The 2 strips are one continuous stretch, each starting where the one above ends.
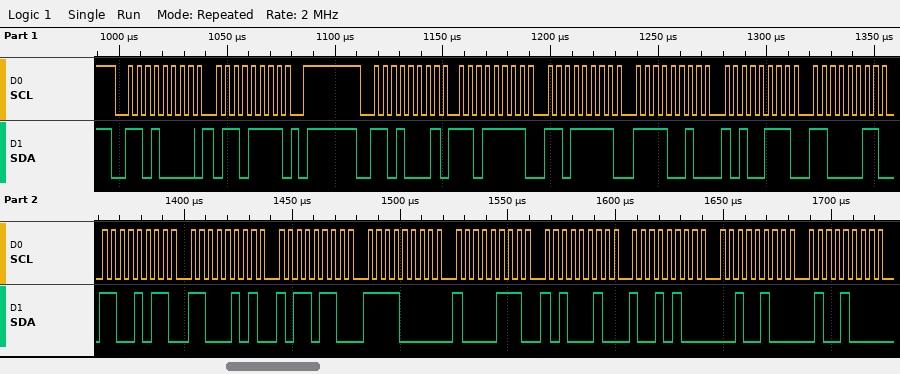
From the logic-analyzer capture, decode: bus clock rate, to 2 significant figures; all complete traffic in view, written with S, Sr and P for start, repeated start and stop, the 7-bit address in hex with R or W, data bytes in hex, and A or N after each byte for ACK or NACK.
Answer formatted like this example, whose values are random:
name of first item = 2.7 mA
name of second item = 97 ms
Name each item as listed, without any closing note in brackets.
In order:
bus clock rate, to 2 significant figures = 250 kHz
all complete traffic in view, written with S, Sr and P for start, repeated start and stop, the 7-bit address in hex with R or W, data bytes in hex, and A or N after each byte for ACK or NACK = S 68W A 6F A P S 68R A DF A DF A F2 A A7 A C3 A CB A C5 A B6 A F0 A 87 A A2 A 94 A 24 A 48 A
